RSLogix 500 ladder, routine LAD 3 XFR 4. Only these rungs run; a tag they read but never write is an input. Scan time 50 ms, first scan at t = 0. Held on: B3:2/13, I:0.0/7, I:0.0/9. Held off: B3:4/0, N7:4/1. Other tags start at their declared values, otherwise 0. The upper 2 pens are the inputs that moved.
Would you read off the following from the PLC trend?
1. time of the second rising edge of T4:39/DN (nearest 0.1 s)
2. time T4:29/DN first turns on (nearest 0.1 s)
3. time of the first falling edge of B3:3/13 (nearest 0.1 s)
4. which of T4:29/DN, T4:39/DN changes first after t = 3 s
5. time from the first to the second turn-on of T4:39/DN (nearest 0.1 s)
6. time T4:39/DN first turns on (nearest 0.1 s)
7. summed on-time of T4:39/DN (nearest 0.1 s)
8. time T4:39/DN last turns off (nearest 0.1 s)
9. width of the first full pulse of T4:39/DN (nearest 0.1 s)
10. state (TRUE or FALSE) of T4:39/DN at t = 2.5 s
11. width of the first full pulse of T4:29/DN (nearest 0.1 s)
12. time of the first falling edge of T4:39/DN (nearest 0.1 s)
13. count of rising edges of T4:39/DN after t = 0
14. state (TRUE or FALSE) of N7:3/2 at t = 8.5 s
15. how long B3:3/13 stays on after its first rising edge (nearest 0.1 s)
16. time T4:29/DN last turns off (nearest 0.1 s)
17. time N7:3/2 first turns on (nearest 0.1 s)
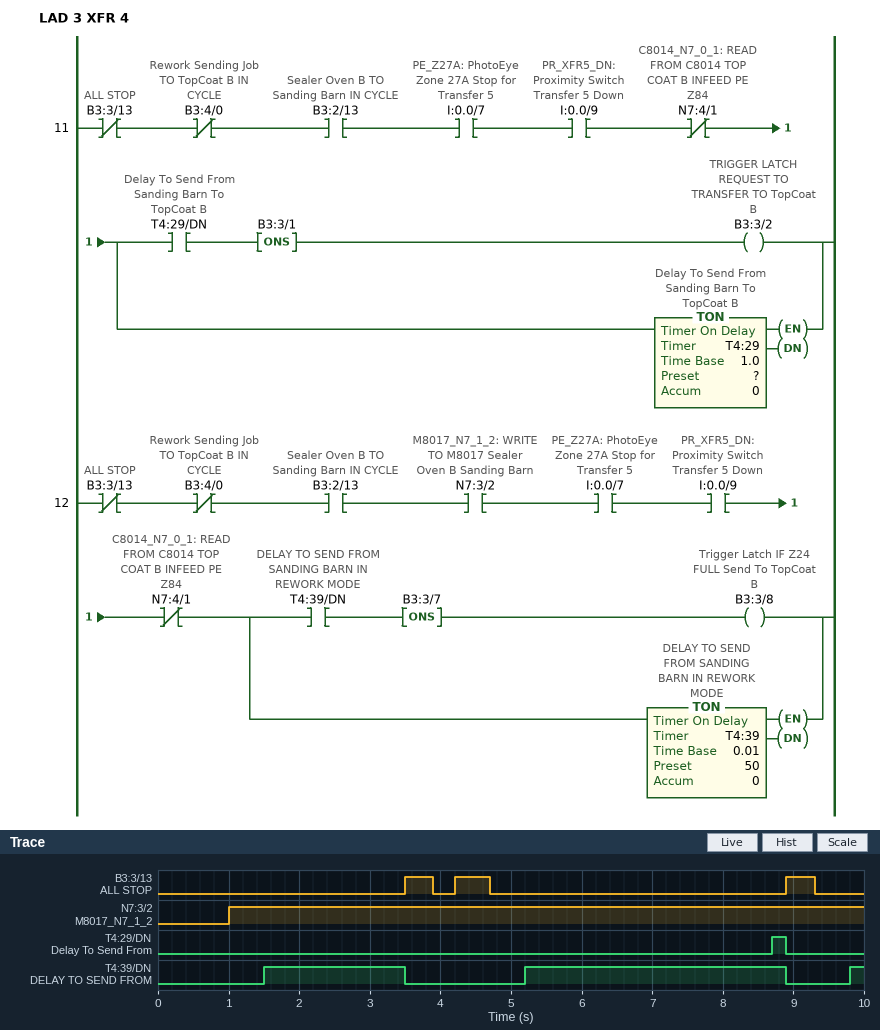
5.2 s
8.7 s
3.9 s
T4:39/DN
3.7 s
1.5 s
5.9 s
8.9 s
2.0 s
TRUE
0.2 s
3.5 s
3
TRUE
0.4 s
8.9 s
1.0 s
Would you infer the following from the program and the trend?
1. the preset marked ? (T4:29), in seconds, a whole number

4 s
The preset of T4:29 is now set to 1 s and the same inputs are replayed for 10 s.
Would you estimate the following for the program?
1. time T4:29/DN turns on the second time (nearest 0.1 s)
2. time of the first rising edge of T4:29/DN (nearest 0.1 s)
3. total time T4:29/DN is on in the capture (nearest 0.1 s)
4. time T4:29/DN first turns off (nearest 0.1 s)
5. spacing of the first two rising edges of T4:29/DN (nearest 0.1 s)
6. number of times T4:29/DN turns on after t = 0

5.7 s
1.0 s
5.7 s
3.5 s
4.7 s
2
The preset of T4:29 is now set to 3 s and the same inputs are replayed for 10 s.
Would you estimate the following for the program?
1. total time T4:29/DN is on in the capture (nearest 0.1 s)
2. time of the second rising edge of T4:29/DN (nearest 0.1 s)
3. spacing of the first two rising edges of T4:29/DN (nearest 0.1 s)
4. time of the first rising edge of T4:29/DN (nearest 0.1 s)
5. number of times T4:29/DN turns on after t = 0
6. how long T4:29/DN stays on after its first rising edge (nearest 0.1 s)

1.7 s
7.7 s
4.7 s
3.0 s
2
0.5 s
